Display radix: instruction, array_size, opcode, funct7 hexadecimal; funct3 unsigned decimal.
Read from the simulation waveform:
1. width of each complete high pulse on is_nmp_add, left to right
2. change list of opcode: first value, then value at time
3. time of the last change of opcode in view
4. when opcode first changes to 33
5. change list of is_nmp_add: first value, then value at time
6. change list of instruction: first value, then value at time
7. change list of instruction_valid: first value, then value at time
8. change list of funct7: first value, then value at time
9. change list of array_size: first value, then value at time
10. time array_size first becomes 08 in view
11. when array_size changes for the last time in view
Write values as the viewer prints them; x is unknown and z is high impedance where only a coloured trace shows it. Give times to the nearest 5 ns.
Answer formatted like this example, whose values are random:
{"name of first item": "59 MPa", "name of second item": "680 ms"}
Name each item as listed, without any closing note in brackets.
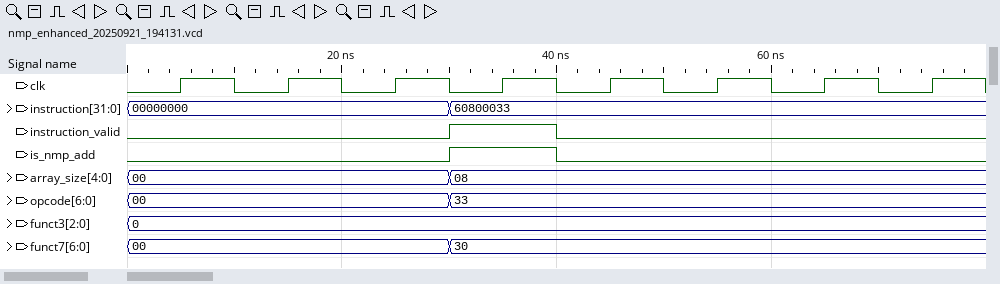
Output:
{"width of each complete high pulse on is_nmp_add, left to right": "10 ns", "change list of opcode: first value, then value at time": "00, 33 at 30 ns", "time of the last change of opcode in view": "30 ns", "when opcode first changes to 33": "30 ns", "change list of is_nmp_add: first value, then value at time": "0, 1 at 30 ns, 0 at 40 ns", "change list of instruction: first value, then value at time": "00000000, 60800033 at 30 ns", "change list of instruction_valid: first value, then value at time": "0, 1 at 30 ns, 0 at 40 ns", "change list of funct7: first value, then value at time": "00, 30 at 30 ns", "change list of array_size: first value, then value at time": "00, 08 at 30 ns", "time array_size first becomes 08 in view": "30 ns", "when array_size changes for the last time in view": "30 ns"}
